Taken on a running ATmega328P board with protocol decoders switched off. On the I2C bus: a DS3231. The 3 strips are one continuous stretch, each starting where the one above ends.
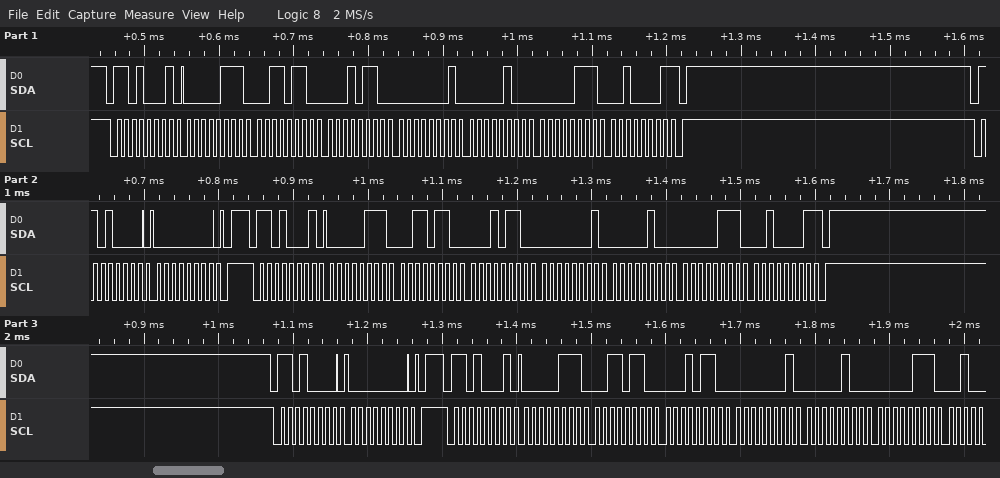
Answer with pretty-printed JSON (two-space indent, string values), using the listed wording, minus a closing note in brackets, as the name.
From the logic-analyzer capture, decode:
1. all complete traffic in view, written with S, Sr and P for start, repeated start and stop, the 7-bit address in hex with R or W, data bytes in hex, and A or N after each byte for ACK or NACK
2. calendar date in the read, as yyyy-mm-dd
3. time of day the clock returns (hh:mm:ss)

{
  "all complete traffic in view, written with S, Sr and P for start, repeated start and stop, the 7-bit address in hex with R or W, data bytes in hex, and A or N after each byte for ACK or NACK": "S 68R A 07 A 36 A 16 A 01 A 04 A 07 A 21 N P S 68W A 00 A P S 68R A 07 A 36 A 16 A 01 A 04 A 07 A 21 N P S 68W A 00 A P S 68R A 07 A 36 A 16 A 01 A 04 A 07 A",
  "calendar date in the read, as yyyy-mm-dd": "2021-07-04",
  "time of day the clock returns": "16:36:07"
}
